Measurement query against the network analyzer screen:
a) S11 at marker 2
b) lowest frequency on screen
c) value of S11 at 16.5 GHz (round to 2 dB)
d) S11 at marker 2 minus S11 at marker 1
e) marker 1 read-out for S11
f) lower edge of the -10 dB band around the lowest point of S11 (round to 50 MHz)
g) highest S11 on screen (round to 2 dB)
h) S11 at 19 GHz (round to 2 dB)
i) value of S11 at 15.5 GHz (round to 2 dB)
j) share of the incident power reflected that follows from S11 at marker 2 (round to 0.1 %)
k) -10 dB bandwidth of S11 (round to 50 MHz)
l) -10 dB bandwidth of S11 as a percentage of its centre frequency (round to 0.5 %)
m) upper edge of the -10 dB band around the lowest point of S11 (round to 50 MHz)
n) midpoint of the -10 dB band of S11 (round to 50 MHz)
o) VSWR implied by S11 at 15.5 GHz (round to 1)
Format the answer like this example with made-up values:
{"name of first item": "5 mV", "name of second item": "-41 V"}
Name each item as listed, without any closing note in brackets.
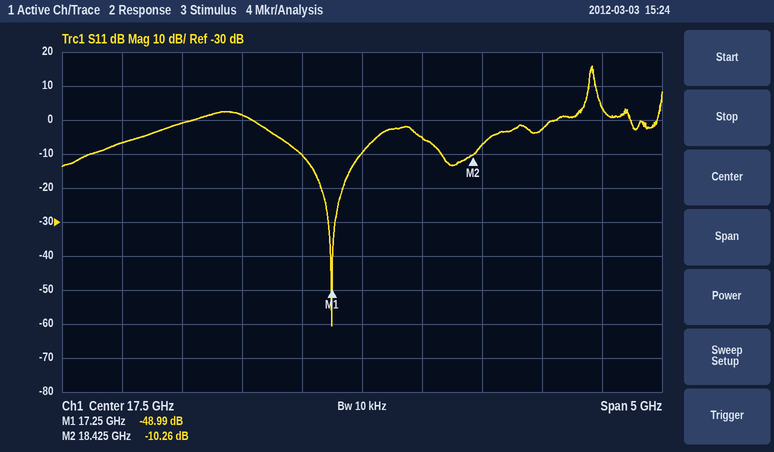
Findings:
{"S11 at marker 2": "-10.26 dB", "lowest frequency on screen": "15 GHz", "value of S11 at 16.5 GHz": "2 dB", "S11 at marker 2 minus S11 at marker 1": "38.73 dB", "marker 1 read-out for S11": "-48.99 dB", "lower edge of the -10 dB band around the lowest point of S11": "17.00 GHz", "highest S11 on screen": "16 dB", "S11 at 19 GHz": "-2 dB", "value of S11 at 15.5 GHz": "-6 dB", "share of the incident power reflected that follows from S11 at marker 2": "9.4 %", "-10 dB bandwidth of S11": "500 MHz", "-10 dB bandwidth of S11 as a percentage of its centre frequency": "3.0 %", "upper edge of the -10 dB band around the lowest point of S11": "17.50 GHz", "midpoint of the -10 dB band of S11": "17.25 GHz", "VSWR implied by S11 at 15.5 GHz": "3"}
